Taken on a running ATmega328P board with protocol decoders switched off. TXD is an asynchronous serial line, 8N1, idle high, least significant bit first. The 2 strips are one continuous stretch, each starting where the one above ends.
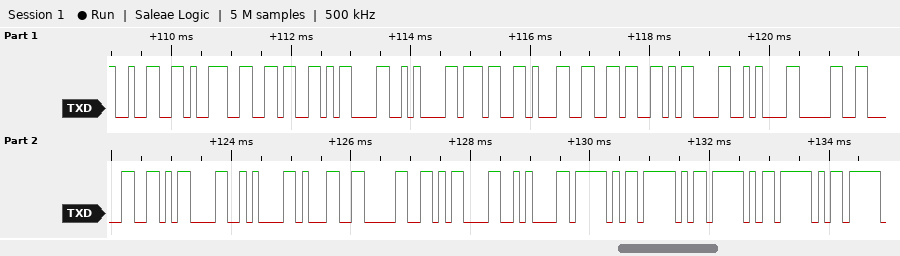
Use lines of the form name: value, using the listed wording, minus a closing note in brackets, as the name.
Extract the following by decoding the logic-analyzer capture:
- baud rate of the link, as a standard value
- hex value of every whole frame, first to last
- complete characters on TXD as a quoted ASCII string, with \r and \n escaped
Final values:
baud rate of the link, as a standard value: 9600 baud
hex value of every whole frame, first to last: 32 39 36 0D 0A 37 31 36 0D 0A 30 30 0D 0A 31 30 0D 0A 5F 5F 5F 5F
complete characters on TXD as a quoted ASCII string, with \r and \n escaped: "296\r\n716\r\n00\r\n10\r\n____"
